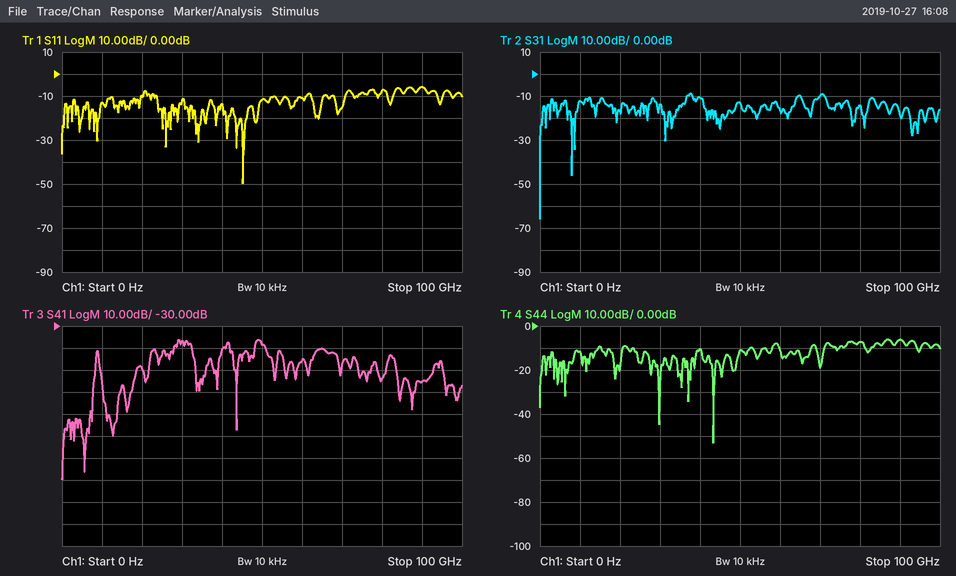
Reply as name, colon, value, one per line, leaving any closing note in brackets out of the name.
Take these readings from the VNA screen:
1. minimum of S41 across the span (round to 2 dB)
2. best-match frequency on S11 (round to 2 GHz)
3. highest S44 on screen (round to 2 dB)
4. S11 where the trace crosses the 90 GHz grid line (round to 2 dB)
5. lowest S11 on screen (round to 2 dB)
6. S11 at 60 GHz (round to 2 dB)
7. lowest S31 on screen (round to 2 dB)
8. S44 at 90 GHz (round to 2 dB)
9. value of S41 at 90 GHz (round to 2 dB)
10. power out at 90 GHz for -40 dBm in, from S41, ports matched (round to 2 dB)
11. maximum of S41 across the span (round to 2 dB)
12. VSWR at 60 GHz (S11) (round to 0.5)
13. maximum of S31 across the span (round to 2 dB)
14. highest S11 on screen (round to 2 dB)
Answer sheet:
minimum of S41 across the span: -100 dB
best-match frequency on S11: 46 GHz
highest S44 on screen: -6 dB
S11 where the trace crosses the 90 GHz grid line: -6 dB
lowest S11 on screen: -50 dB
S11 at 60 GHz: -10 dB
lowest S31 on screen: -66 dB
S44 at 90 GHz: -6 dB
value of S41 at 90 GHz: -56 dB
power out at 90 GHz for -40 dBm in, from S41, ports matched: -96 dBm
maximum of S41 across the span: -36 dB
VSWR at 60 GHz (S11): 2.0
maximum of S31 across the span: -8 dB
highest S11 on screen: -6 dB
